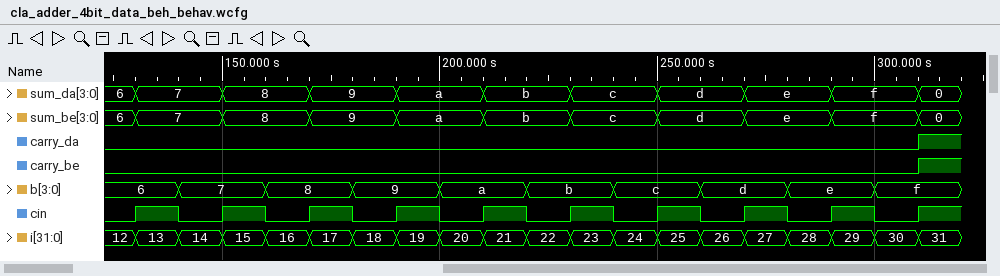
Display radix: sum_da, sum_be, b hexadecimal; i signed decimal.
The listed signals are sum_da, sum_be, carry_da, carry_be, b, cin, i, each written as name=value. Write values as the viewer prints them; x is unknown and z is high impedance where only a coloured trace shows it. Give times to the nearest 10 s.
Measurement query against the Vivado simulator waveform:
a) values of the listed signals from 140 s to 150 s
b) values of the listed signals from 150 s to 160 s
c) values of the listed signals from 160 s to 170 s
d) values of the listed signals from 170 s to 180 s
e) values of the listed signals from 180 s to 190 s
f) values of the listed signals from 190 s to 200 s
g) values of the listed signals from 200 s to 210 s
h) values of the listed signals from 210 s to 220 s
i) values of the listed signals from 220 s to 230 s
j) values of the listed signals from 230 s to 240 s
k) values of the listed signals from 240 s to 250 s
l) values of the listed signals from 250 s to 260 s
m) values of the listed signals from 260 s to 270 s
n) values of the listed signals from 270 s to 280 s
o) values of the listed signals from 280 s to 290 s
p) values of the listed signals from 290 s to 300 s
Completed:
sum_da=7, sum_be=7, carry_da=0, carry_be=0, b=7, cin=0, i=14
sum_da=8, sum_be=8, carry_da=0, carry_be=0, b=7, cin=1, i=15
sum_da=8, sum_be=8, carry_da=0, carry_be=0, b=8, cin=0, i=16
sum_da=9, sum_be=9, carry_da=0, carry_be=0, b=8, cin=1, i=17
sum_da=9, sum_be=9, carry_da=0, carry_be=0, b=9, cin=0, i=18
sum_da=a, sum_be=a, carry_da=0, carry_be=0, b=9, cin=1, i=19
sum_da=a, sum_be=a, carry_da=0, carry_be=0, b=a, cin=0, i=20
sum_da=b, sum_be=b, carry_da=0, carry_be=0, b=a, cin=1, i=21
sum_da=b, sum_be=b, carry_da=0, carry_be=0, b=b, cin=0, i=22
sum_da=c, sum_be=c, carry_da=0, carry_be=0, b=b, cin=1, i=23
sum_da=c, sum_be=c, carry_da=0, carry_be=0, b=c, cin=0, i=24
sum_da=d, sum_be=d, carry_da=0, carry_be=0, b=c, cin=1, i=25
sum_da=d, sum_be=d, carry_da=0, carry_be=0, b=d, cin=0, i=26
sum_da=e, sum_be=e, carry_da=0, carry_be=0, b=d, cin=1, i=27
sum_da=e, sum_be=e, carry_da=0, carry_be=0, b=e, cin=0, i=28
sum_da=f, sum_be=f, carry_da=0, carry_be=0, b=e, cin=1, i=29
